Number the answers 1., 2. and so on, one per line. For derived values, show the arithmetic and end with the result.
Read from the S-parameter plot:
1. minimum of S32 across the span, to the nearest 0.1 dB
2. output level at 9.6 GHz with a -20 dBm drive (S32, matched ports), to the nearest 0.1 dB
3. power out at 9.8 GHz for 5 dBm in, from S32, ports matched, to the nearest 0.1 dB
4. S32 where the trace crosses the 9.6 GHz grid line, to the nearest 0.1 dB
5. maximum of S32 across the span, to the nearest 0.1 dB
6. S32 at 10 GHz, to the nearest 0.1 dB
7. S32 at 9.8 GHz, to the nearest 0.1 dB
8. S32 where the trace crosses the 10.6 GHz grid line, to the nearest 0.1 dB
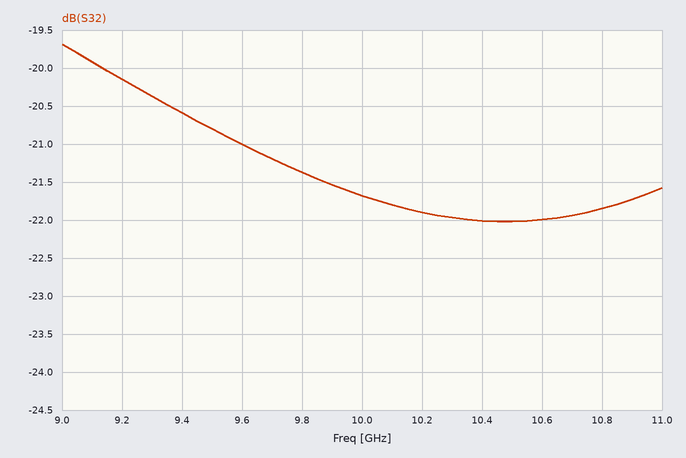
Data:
1. -22.0 dB
2. -20 dBm + (-21.0 dB) = -41.0 dBm
3. 5 dBm + (-21.4 dB) = -16.4 dBm
4. -21.0 dB
5. -19.7 dB
6. -21.7 dB
7. -21.4 dB
8. -22.0 dB
